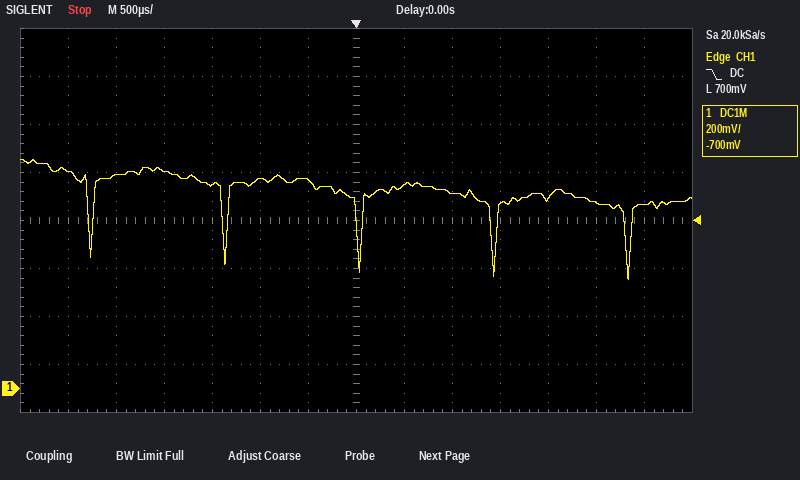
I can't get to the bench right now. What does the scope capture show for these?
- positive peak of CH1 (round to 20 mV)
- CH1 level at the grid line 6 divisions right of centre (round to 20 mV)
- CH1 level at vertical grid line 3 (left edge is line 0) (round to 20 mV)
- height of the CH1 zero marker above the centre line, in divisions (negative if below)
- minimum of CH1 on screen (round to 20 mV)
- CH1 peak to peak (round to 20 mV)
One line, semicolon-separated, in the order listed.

960 mV; 760 mV; 900 mV; -3.5 div; 460 mV; 500 mV
